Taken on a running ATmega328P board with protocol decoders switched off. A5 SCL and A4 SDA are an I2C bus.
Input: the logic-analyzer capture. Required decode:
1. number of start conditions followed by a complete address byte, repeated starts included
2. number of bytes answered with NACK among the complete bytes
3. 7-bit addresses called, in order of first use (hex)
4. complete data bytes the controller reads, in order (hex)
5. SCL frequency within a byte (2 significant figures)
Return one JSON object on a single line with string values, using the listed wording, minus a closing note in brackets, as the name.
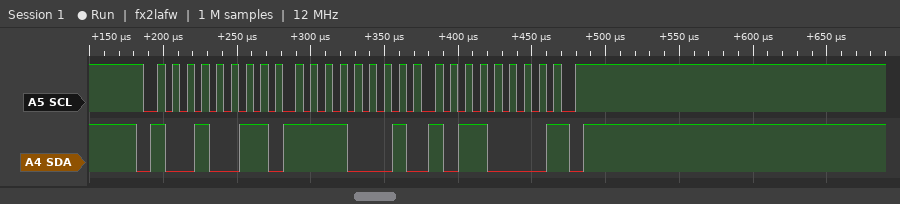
{"number of start conditions followed by a complete address byte, repeated starts included": "1", "number of bytes answered with NACK among the complete bytes": "1", "7-bit addresses called, in order of first use": "0x49", "complete data bytes the controller reads, in order": "F1 B0", "SCL frequency within a byte": "100 kHz"}
